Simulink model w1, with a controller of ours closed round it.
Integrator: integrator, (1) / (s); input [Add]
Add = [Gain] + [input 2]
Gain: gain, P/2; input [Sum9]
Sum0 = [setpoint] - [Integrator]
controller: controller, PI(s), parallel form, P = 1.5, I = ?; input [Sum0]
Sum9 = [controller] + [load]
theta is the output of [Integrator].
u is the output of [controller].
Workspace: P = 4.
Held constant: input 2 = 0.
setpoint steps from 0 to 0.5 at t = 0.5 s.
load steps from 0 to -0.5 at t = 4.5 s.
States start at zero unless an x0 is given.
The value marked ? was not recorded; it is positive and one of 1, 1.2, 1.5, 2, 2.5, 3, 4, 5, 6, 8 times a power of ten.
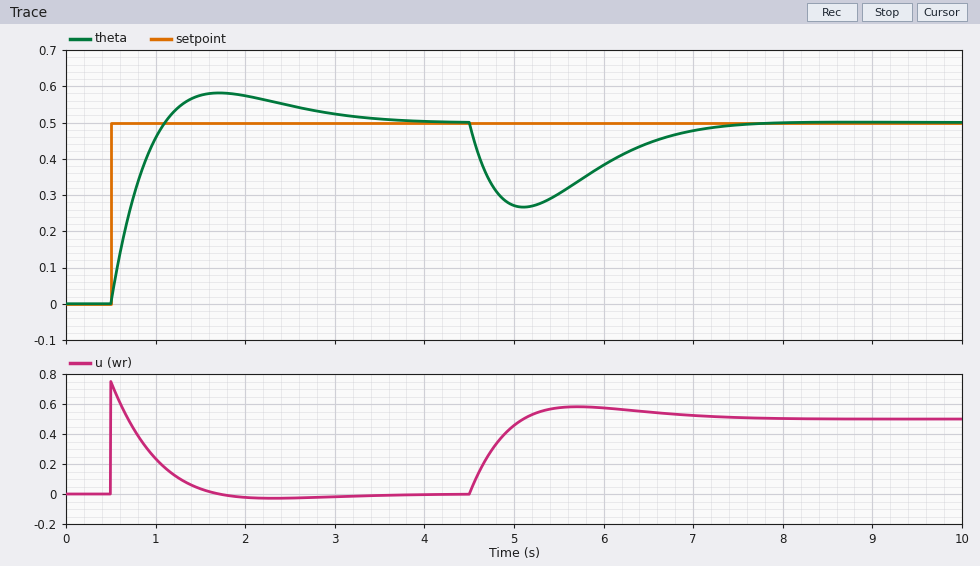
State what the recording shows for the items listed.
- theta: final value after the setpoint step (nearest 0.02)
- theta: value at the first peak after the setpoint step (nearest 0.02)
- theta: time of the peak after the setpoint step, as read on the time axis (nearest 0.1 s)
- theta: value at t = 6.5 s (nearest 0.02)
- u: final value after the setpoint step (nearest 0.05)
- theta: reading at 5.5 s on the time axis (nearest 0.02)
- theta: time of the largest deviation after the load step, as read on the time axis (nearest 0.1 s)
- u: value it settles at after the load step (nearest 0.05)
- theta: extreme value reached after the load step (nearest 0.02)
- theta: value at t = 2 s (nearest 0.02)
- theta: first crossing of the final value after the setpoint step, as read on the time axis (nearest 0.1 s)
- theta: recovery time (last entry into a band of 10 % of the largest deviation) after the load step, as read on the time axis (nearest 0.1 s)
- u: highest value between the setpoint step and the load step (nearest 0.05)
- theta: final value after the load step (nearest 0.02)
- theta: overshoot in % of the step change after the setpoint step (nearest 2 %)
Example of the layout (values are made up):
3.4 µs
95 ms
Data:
0.50
0.58
1.7 s
0.44
0.00
0.30
5.1 s
0.50
0.26
0.58
1.1 s
7.0 s
0.75
0.50
16 %
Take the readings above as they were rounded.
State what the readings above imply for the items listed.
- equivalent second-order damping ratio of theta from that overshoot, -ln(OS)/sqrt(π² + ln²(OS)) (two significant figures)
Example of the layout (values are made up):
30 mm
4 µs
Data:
0.50
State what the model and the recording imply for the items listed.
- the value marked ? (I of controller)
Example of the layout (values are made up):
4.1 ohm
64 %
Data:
1.5
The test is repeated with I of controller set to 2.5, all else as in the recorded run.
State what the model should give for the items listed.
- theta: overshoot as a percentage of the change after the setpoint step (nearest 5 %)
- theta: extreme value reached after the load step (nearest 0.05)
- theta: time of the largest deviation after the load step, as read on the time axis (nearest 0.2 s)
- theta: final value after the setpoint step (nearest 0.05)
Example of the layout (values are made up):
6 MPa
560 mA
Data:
20 %
0.30
5.0 s
0.50
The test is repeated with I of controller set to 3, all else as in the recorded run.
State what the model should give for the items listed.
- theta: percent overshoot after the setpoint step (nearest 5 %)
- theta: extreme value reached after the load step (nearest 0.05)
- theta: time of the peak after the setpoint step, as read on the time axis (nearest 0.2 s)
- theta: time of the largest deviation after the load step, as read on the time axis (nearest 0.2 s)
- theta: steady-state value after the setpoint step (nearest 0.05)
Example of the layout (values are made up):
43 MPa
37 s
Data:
25 %
0.30
1.4 s
5.0 s
0.50
